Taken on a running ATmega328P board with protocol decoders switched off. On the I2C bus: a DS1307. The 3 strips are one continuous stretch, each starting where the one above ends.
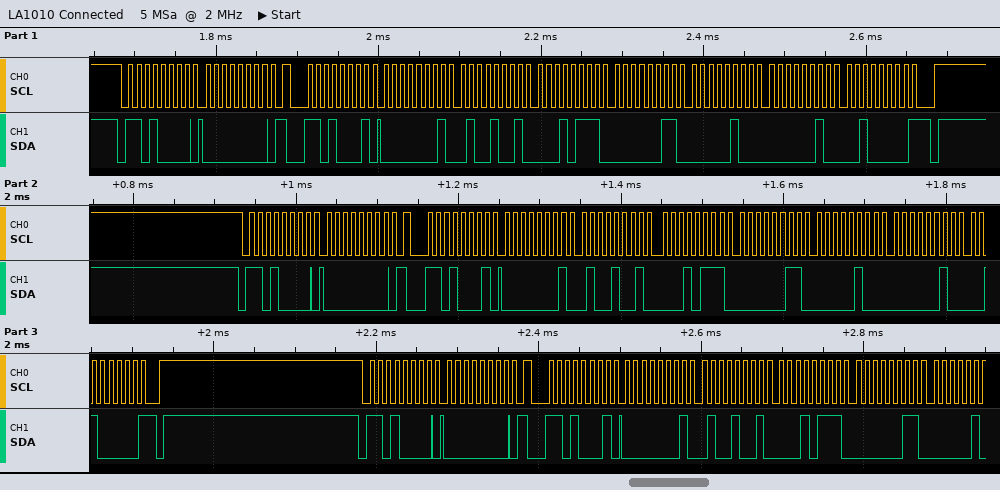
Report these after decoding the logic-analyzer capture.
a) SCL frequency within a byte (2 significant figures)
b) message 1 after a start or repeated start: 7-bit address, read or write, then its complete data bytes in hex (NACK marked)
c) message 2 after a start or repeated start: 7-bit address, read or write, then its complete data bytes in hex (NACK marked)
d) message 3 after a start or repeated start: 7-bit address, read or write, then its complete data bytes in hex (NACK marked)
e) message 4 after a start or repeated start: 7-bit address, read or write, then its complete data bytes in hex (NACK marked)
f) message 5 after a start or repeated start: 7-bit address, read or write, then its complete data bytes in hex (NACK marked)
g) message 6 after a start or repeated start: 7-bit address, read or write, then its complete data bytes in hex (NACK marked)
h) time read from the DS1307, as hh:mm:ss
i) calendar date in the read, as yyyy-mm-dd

100 kHz
0x68 write: 00
0x68 read: 01 49 17 03 04 02 20 NACK
0x68 write: 00
0x68 read: 01 49 17 03 04 02 20 NACK
0x68 write: 00
0x68 read: 01 49 17 03
17:49:01
2020-02-04
